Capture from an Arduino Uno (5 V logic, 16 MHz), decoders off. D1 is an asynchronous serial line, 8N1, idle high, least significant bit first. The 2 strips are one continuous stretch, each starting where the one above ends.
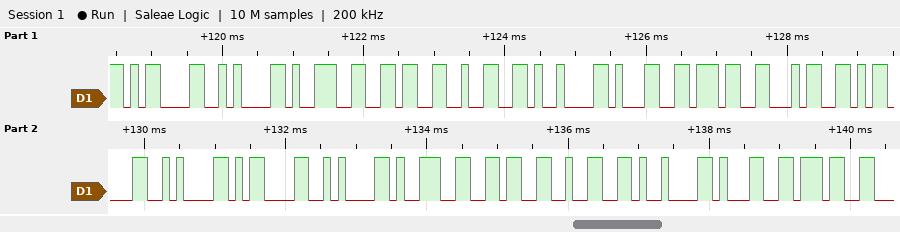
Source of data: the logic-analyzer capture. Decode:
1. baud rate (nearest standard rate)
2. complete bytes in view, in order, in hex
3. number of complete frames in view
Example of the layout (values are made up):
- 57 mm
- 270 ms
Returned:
- 9600 baud
- 0x0D 0x0A 0x39 0x36 0x32 0x09 0x31 0x37 0x34 0x0D 0x0A 0x0D 0x0A 0x39 0x36 0x32 0x09 0x31 0x37
- 19
